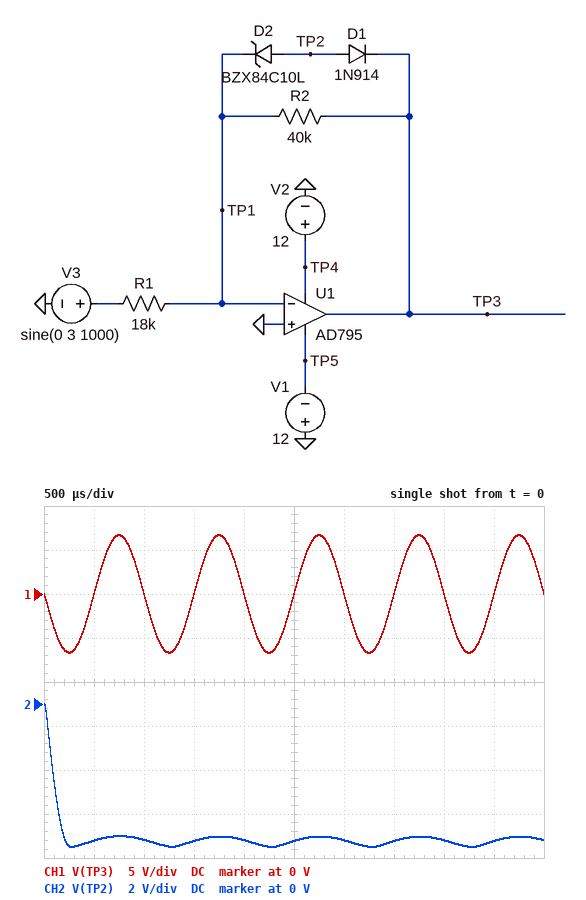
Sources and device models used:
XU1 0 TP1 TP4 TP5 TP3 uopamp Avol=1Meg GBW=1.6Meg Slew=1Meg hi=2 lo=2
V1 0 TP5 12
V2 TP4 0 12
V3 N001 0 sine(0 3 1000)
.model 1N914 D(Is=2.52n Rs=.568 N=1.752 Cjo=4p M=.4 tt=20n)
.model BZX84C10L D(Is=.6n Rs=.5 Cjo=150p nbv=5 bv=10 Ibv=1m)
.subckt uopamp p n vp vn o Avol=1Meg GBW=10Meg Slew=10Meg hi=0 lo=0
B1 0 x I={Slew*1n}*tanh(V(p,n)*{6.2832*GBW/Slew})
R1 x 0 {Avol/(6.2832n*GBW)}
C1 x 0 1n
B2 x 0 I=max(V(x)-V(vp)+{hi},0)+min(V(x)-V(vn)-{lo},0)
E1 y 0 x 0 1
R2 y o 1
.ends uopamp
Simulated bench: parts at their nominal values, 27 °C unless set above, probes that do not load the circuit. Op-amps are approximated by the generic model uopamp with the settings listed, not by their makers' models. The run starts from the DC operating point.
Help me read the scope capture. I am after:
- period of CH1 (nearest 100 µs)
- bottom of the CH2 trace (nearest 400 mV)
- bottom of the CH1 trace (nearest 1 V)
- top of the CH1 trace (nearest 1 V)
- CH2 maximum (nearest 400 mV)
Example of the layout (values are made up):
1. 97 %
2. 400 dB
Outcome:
1. 1.0 ms
2. -6.4 V
3. -7 V
4. 7 V
5. 0 V
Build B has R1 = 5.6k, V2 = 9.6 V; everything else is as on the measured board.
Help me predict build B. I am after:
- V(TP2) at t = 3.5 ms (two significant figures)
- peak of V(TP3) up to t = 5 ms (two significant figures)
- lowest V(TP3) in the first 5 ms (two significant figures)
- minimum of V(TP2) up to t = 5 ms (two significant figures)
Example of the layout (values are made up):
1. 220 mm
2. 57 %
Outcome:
1. -8.5 V
2. 7.6 V
3. -10 V
4. -9.9 V
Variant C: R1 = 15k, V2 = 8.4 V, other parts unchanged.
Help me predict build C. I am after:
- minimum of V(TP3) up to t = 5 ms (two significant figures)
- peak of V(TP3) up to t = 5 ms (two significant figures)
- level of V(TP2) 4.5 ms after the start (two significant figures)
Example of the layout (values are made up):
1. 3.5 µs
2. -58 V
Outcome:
1. -8.0 V
2. 6.4 V
3. -7.5 V
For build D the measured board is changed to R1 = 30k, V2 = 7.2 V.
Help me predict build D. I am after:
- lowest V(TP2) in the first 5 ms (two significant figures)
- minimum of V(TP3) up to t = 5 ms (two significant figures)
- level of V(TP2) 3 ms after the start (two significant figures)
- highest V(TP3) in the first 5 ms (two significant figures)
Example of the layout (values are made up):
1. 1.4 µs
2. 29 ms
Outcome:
1. -3.9 V
2. -4.0 V
3. -3.7 V
4. 4.0 V
